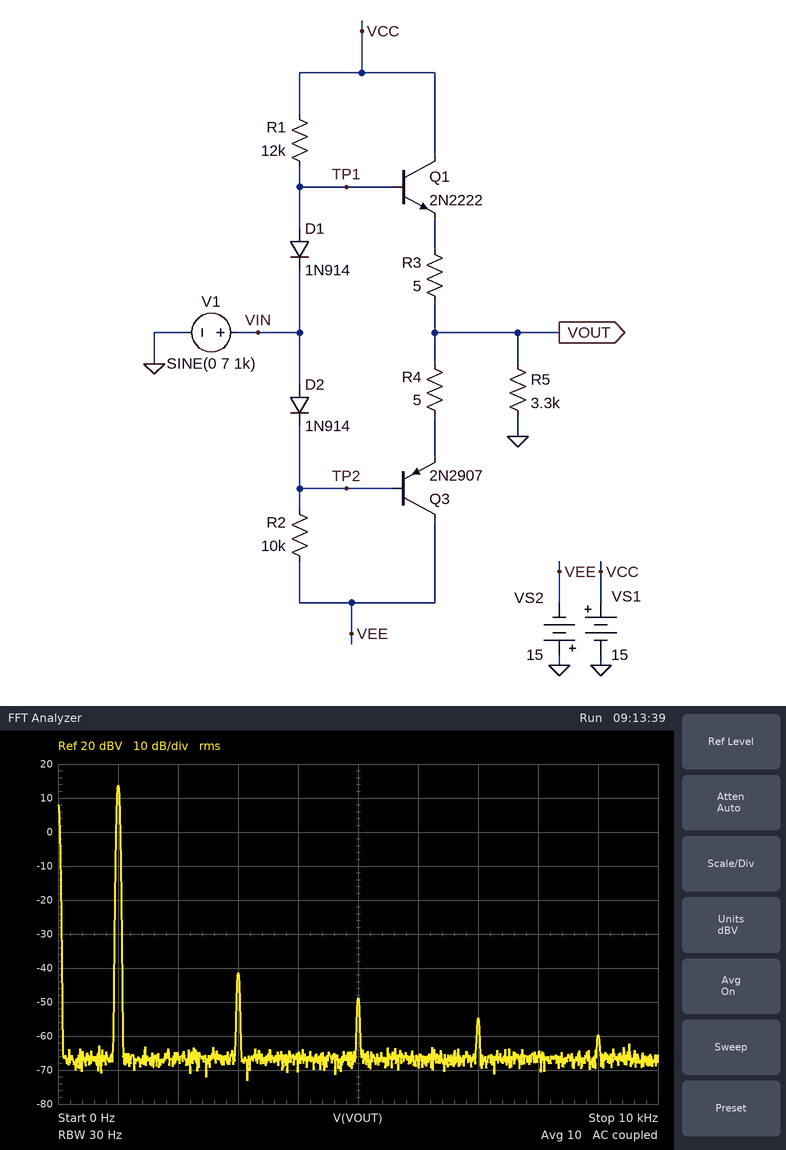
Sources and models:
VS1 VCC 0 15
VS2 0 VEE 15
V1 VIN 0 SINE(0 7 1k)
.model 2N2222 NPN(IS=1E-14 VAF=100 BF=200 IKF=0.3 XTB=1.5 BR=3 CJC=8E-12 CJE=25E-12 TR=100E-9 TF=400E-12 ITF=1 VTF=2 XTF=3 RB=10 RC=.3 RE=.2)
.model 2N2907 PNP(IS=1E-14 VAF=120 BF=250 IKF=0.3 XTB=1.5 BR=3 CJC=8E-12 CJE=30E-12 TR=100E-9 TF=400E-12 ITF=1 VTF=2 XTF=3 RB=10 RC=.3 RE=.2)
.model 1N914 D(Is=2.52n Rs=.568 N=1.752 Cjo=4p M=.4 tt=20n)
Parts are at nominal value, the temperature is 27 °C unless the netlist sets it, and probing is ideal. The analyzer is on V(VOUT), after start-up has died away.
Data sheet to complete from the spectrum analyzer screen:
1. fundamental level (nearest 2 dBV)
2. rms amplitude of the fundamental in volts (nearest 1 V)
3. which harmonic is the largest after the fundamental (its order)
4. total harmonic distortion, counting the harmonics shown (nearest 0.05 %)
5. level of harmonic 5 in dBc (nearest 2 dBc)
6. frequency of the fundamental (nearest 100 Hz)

14 dBV
5 V
3
0.20 %
-62 dBc
1.0 kHz
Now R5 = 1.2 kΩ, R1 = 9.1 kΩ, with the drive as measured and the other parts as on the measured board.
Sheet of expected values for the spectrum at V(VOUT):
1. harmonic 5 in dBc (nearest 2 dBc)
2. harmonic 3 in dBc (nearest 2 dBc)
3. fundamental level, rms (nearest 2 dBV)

-58 dBc
-50 dBc
14 dBV
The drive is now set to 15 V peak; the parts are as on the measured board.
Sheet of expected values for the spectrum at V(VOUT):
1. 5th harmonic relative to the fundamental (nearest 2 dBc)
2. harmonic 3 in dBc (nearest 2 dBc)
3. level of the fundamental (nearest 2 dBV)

-40 dBc
-38 dBc
20 dBV
